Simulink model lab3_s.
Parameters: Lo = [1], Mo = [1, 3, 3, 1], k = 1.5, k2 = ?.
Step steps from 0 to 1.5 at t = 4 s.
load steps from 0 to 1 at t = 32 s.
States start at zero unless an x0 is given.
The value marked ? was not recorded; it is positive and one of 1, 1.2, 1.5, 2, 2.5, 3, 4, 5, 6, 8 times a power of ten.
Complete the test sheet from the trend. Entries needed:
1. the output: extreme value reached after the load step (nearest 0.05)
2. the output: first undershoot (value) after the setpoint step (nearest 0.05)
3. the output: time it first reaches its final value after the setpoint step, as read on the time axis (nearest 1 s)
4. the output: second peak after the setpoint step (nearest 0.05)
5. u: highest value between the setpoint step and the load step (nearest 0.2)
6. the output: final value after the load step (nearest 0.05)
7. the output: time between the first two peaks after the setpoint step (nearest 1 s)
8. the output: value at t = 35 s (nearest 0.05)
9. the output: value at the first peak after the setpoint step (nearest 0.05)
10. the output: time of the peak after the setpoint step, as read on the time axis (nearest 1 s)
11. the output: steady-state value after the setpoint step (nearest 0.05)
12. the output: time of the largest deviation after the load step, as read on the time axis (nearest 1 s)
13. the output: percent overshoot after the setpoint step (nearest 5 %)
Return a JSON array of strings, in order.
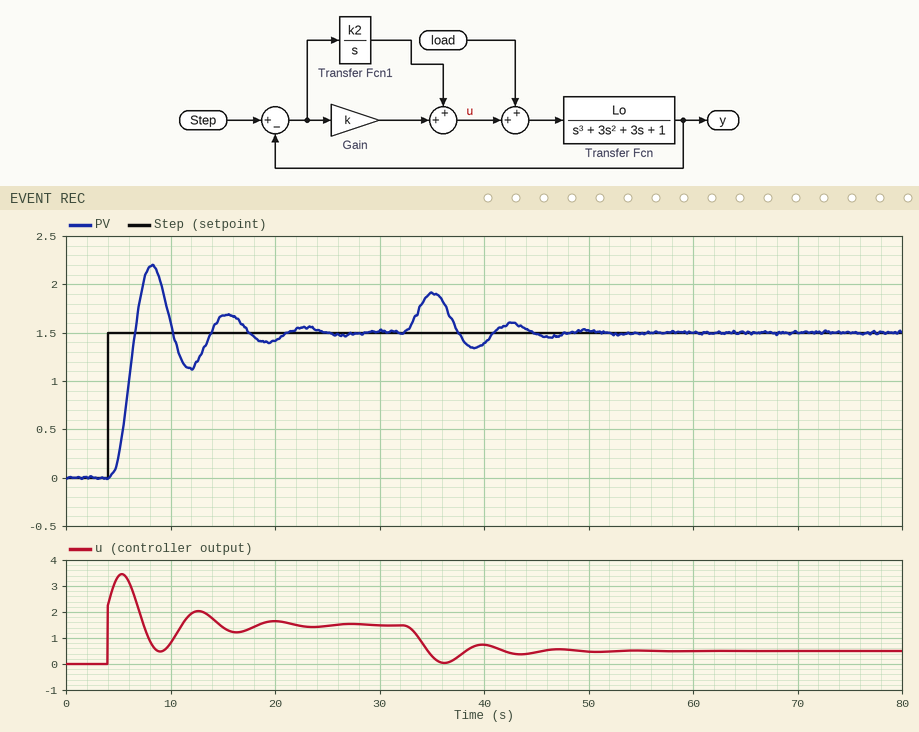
["1.90", "1.15", "7 s", "1.70", "3.4", "1.50", "7 s", "1.90", "2.20", "8 s", "1.50", "35 s", "45 %"]
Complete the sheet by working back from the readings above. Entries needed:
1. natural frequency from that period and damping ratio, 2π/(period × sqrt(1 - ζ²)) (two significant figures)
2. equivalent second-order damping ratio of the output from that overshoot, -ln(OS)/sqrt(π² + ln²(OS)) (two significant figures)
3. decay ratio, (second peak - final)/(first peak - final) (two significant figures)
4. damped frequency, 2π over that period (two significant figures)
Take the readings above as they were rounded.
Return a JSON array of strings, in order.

["0.93 rad/s", "0.25", "0.29", "0.90 rad/s"]
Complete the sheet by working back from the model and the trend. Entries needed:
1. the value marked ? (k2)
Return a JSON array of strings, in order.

["1"]
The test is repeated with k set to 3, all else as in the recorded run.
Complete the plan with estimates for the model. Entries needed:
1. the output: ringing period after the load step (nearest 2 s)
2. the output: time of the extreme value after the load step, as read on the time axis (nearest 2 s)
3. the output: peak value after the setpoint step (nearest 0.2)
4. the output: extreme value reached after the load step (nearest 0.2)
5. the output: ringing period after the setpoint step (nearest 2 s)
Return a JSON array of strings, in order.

["6 s", "34 s", "2.2", "1.8", "6 s"]
